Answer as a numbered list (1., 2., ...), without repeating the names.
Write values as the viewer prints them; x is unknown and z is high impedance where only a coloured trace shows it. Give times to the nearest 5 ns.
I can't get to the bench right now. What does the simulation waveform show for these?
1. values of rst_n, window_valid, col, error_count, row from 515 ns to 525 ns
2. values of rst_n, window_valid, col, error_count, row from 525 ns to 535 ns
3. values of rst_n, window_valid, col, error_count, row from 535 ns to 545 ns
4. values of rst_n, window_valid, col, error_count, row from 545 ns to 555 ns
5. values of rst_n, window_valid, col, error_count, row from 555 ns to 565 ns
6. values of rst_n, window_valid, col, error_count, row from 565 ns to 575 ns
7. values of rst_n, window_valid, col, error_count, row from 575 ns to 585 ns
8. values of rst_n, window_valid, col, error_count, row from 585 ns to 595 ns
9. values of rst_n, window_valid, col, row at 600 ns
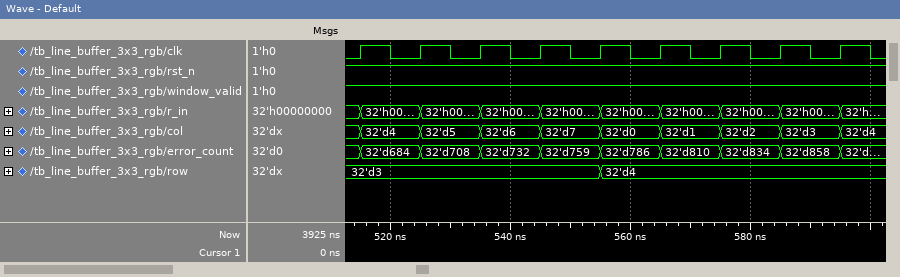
1. rst_n=1, window_valid=1, col=32'd4, error_count=32'd684, row=32'd3
2. rst_n=1, window_valid=1, col=32'd5, error_count=32'd708, row=32'd3
3. rst_n=1, window_valid=1, col=32'd6, error_count=32'd732, row=32'd3
4. rst_n=1, window_valid=1, col=32'd7, error_count=32'd759, row=32'd3
5. rst_n=1, window_valid=1, col=32'd0, error_count=32'd786, row=32'd4
6. rst_n=1, window_valid=1, col=32'd1, error_count=32'd810, row=32'd4
7. rst_n=1, window_valid=1, col=32'd2, error_count=32'd834, row=32'd4
8. rst_n=1, window_valid=1, col=32'd3, error_count=32'd858, row=32'd4
9. rst_n=1, window_valid=1, col=32'd4, row=32'd4
